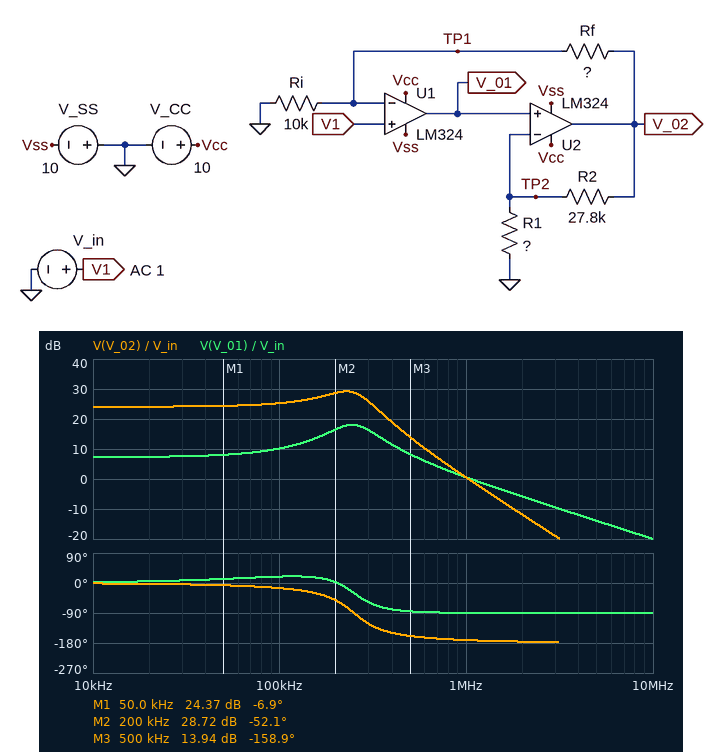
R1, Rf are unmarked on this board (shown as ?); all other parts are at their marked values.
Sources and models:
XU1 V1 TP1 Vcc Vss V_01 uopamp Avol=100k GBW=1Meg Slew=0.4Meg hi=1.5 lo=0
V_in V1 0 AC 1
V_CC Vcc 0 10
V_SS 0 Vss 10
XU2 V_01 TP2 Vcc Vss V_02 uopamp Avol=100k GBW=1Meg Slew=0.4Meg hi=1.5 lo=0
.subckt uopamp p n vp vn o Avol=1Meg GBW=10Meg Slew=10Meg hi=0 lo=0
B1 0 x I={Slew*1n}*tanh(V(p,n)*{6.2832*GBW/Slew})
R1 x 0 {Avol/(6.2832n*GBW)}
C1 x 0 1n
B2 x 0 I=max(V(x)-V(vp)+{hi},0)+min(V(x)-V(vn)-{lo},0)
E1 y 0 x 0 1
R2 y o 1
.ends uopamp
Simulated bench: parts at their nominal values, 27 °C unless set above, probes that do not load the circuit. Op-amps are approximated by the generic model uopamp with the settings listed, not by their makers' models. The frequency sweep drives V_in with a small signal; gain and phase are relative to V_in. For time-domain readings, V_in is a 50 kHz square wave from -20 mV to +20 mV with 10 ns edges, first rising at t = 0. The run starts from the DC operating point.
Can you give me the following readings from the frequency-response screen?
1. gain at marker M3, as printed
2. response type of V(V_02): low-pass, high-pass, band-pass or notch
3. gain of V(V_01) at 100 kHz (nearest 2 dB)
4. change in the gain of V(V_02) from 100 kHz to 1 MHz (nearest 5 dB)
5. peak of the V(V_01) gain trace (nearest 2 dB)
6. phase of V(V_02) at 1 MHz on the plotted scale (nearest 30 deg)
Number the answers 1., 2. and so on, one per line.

1. 13.94 dB
2. low-pass
3. 10 dB
4. -25 dB
5. 18 dB
6. -180 deg
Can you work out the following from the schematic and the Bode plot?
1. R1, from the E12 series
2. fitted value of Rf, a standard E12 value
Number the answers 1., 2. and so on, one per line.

1. 4.7 kΩ
2. 150 kΩ
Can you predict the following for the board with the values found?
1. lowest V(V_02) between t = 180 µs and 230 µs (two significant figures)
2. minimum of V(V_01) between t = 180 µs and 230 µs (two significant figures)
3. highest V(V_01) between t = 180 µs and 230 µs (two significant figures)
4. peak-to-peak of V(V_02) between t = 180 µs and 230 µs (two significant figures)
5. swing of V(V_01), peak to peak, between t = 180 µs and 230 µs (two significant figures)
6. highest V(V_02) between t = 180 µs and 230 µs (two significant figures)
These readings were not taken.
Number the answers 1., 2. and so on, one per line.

1. -660 mV
2. -190 mV
3. 190 mV
4. 1.3 V
5. 370 mV
6. 660 mV
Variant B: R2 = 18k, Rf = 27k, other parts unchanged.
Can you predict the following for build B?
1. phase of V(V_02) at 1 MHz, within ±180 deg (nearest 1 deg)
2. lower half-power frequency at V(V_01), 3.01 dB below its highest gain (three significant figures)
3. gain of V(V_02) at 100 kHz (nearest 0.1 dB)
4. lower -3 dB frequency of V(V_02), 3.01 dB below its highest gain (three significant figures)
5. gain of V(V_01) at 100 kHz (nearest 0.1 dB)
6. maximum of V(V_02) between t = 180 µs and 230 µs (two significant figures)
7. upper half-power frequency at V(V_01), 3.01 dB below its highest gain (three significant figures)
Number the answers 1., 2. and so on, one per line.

1. -164 deg
2. 421 kHz
3. 11.7 dB
4. 379 kHz
5. -1.1 dB
6. 160 mV
7. 628 kHz
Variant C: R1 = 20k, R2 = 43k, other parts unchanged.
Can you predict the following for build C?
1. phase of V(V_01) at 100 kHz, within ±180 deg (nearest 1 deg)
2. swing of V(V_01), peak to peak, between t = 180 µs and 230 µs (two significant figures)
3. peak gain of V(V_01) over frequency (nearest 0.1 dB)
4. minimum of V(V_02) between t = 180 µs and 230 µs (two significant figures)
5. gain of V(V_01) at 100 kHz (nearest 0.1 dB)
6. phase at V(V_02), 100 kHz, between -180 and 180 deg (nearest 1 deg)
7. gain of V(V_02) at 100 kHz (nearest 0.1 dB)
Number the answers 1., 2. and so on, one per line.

1. -14 deg
2. 310 mV
3. 15.1 dB
4. -420 mV
5. 14.7 dB
6. -31 deg
7. 24.2 dB
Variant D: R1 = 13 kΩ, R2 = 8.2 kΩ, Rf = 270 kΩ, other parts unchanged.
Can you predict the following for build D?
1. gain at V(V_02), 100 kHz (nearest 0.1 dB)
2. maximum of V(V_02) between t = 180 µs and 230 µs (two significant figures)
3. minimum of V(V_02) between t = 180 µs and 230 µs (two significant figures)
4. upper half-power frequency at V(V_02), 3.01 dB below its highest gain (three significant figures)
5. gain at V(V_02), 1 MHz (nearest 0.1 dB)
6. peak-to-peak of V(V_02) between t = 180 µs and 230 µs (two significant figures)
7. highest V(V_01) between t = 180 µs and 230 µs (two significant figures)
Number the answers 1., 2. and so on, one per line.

1. 23.5 dB
2. 540 mV
3. -540 mV
4. 64.3 kHz
5. -1.2 dB
6. 1.1 V
7. 330 mV
